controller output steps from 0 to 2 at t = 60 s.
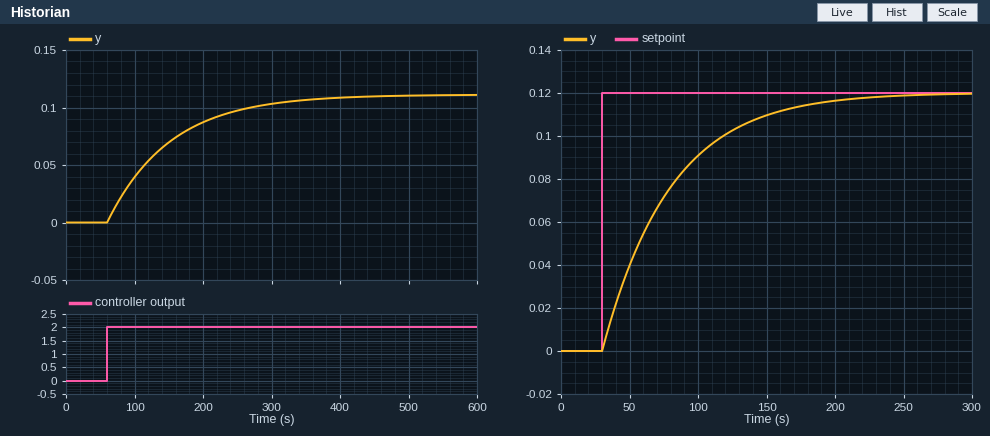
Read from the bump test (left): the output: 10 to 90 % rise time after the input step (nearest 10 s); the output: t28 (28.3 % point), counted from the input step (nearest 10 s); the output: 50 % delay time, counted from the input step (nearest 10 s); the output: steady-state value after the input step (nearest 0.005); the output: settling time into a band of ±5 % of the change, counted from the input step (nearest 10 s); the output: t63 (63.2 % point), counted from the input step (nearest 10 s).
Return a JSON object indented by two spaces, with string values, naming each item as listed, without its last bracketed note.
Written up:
{
  "the output: 10 to 90 % rise time after the input step": "200 s",
  "the output: t28 (28.3 % point), counted from the input step": "30 s",
  "the output: 50 % delay time, counted from the input step": "60 s",
  "the output: steady-state value after the input step": "0.110",
  "the output: settling time into a band of ±5 % of the change, counted from the input step": "270 s",
  "the output: t63 (63.2 % point), counted from the input step": "90 s"
}
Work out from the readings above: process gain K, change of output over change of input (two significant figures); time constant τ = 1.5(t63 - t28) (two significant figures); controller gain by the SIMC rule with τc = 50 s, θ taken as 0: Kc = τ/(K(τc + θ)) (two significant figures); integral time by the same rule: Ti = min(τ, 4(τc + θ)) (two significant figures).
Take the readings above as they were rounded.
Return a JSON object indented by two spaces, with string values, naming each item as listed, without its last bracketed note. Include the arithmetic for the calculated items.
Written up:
{
  "process gain K, change of output over change of input": "(0.11 - 0) / 2 = 0.055",
  "time constant τ = 1.5(t63 - t28)": "1.5 × (90 - 30) = 90 s",
  "controller gain by the SIMC rule with τc = 50 s, θ taken as 0: Kc = τ/(K(τc + θ))": "90 / (0.055 × (50 + 0)) = 33",
  "integral time by the same rule: Ti = min(τ, 4(τc + θ))": "min(90, 4 × (50 + 0)) = 90 s"
}
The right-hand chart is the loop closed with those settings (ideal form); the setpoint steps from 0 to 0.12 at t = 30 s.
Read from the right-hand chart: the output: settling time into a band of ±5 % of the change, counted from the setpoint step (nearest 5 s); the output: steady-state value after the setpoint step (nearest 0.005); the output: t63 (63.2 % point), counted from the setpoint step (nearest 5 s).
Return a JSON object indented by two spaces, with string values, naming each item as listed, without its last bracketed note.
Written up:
{
  "the output: settling time into a band of ±5 % of the change, counted from the setpoint step": "145 s",
  "the output: steady-state value after the setpoint step": "0.120",
  "the output: t63 (63.2 % point), counted from the setpoint step": "50 s"
}
